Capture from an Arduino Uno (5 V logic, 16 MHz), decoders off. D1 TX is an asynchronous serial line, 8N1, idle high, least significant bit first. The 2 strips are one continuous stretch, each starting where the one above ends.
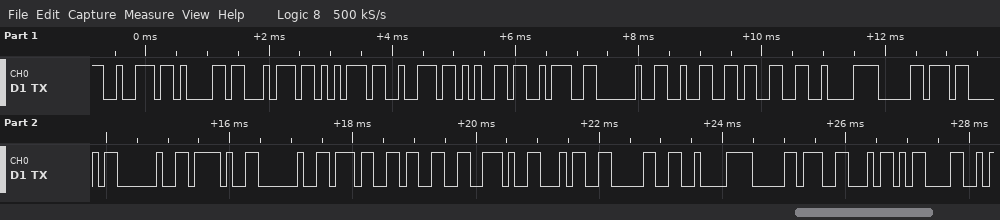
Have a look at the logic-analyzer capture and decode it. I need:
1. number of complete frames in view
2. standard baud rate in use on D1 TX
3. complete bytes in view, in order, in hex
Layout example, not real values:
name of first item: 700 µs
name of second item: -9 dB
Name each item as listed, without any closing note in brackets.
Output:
number of complete frames in view: 25
standard baud rate in use on D1 TX: 9600 baud
complete bytes in view, in order, in hex: 72 61 74 75 72 65 3A 20 32 33 C2 B0 43 20 2F 20 37 33 2E 34 30 C2 B0 46 0D
